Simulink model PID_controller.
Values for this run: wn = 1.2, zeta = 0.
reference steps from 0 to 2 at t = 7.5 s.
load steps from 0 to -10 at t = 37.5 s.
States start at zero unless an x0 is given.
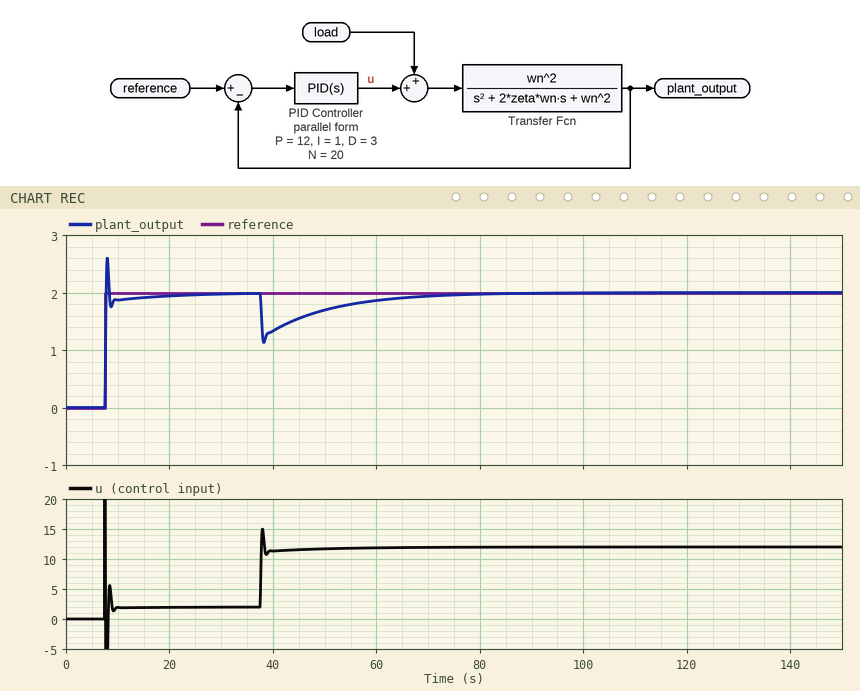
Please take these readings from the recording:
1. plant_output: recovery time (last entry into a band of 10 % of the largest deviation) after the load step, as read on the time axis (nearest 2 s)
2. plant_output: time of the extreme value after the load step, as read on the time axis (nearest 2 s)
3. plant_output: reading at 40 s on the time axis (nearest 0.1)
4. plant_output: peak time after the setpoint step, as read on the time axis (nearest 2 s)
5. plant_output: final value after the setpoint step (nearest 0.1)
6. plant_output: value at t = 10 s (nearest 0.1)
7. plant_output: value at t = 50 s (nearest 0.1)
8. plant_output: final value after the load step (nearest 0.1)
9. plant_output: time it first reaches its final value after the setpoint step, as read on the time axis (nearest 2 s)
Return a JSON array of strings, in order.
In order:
["66 s", "38 s", "1.3", "8 s", "2.0", "1.9", "1.7", "2.0", "8 s"]
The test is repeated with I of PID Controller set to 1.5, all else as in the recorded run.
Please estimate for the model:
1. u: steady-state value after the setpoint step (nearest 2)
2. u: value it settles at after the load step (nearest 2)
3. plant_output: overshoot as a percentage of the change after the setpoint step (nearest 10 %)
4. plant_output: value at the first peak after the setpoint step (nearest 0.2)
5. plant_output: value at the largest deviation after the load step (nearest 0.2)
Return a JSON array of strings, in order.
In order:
["2", "12", "30 %", "2.6", "1.2"]
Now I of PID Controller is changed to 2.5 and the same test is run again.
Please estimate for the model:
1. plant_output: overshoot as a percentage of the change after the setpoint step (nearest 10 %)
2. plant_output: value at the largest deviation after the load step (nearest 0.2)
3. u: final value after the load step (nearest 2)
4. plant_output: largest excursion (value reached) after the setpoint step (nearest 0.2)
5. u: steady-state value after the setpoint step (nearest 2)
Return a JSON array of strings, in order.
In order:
["30 %", "1.2", "12", "2.6", "2"]
